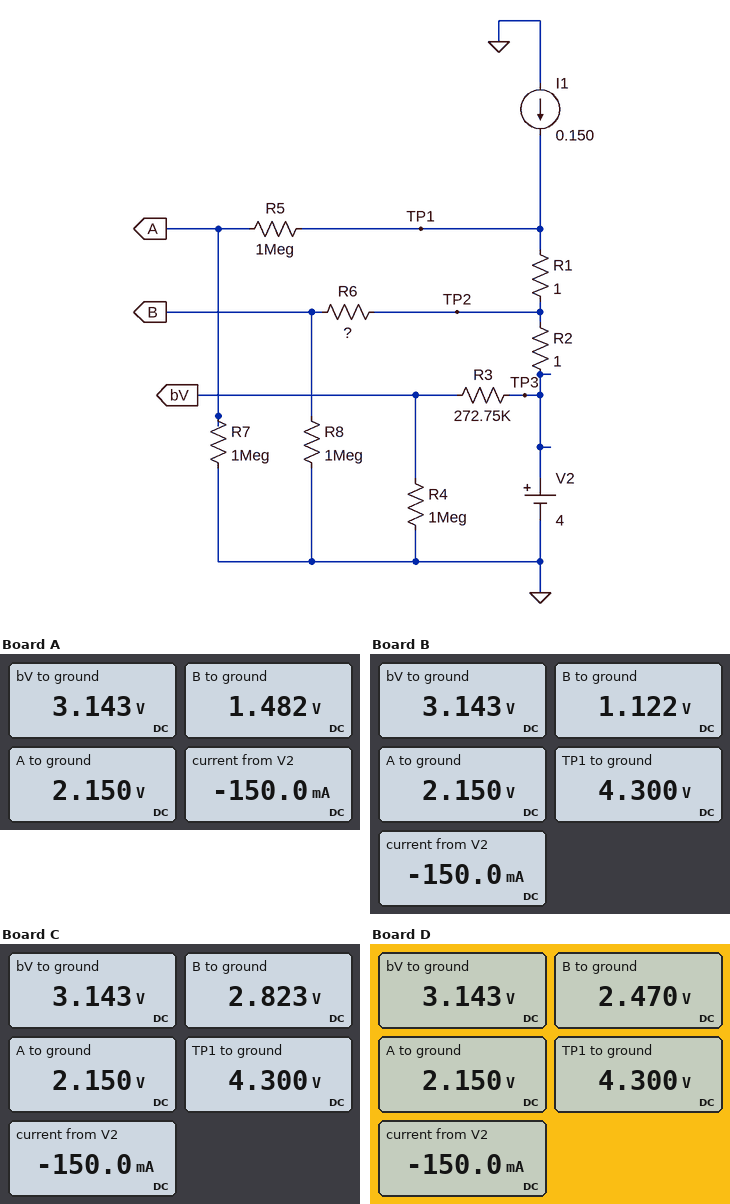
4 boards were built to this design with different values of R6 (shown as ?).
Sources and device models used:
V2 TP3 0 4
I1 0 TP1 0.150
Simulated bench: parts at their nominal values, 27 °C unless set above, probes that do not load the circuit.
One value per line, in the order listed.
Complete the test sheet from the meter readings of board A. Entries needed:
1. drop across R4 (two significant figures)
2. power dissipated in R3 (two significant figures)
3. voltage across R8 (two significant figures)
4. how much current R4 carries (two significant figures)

3.1 V
2.7 µW
1.5 V
3.1 µA
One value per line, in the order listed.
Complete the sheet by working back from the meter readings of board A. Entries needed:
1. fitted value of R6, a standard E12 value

1.8 MΩ
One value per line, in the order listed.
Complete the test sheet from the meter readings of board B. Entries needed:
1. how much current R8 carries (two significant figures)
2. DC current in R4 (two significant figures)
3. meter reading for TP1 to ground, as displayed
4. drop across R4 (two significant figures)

1.1 µA
3.1 µA
4.300 V
3.1 V
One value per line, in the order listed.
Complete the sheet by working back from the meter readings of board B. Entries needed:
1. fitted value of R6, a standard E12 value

2.7 MΩ
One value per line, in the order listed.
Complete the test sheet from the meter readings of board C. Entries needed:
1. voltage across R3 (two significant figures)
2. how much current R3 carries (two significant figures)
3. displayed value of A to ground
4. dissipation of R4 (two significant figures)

860 mV
3.1 µA
2.150 V
9.9 µW
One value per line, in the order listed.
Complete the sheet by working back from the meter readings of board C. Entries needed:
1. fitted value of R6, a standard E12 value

470 kΩ
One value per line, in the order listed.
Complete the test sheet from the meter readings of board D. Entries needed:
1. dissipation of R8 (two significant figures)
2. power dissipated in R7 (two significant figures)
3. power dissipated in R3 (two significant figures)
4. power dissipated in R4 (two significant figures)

6.1 µW
4.6 µW
2.7 µW
9.9 µW
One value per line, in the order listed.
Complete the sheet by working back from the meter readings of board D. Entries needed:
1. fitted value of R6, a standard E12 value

680 kΩ
